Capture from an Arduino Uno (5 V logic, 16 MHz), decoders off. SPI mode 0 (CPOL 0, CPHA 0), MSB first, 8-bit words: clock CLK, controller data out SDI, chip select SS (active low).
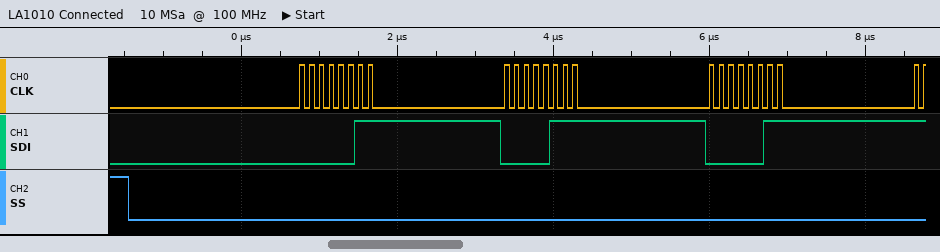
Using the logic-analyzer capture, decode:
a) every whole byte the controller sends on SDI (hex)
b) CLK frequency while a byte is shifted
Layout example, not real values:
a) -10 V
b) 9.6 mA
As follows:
a) 03 07 03
b) 8 MHz
